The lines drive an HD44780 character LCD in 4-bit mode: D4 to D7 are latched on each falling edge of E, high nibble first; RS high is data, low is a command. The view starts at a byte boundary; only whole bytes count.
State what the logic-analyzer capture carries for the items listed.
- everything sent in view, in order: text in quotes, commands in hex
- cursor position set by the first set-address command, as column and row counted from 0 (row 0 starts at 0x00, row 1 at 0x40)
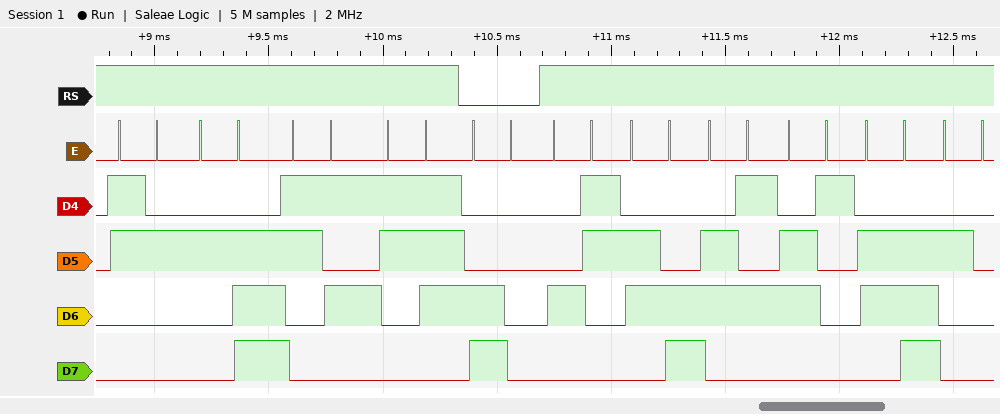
"2.57" 0xC0 "Clean "
column 0, row 1
